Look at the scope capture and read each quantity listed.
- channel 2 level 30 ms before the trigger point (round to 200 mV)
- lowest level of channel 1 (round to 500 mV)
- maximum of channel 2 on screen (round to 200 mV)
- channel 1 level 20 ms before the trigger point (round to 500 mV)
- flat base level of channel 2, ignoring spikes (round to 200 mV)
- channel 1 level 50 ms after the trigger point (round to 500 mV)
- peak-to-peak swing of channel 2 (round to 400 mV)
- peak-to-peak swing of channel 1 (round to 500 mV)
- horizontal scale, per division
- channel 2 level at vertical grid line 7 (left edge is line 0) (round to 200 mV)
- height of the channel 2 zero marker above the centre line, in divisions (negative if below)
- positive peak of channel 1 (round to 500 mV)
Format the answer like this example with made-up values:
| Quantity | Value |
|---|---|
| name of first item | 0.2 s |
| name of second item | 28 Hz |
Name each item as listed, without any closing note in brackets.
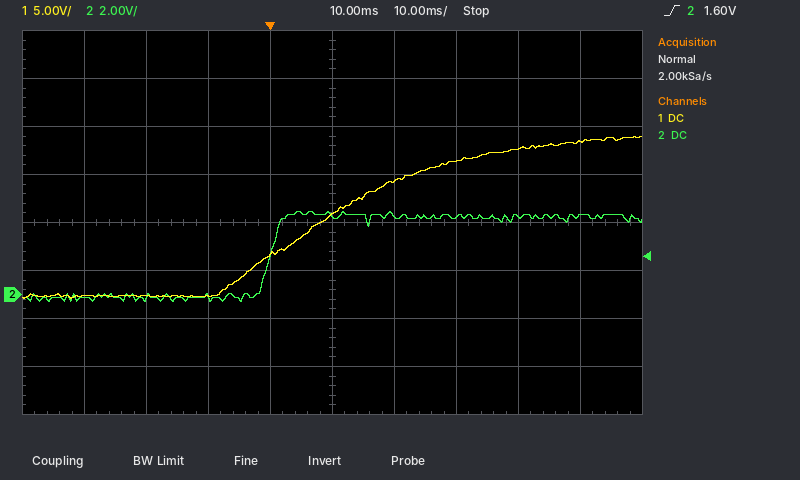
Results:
| Quantity | Value |
|---|---|
| channel 2 level 30 ms before the trigger point | -200 mV |
| lowest level of channel 1 | -500 mV |
| maximum of channel 2 on screen | 3.4 V |
| channel 1 level 20 ms before the trigger point | 0.0 V |
| flat base level of channel 2, ignoring spikes | -200 mV |
| channel 1 level 50 ms after the trigger point | 16.0 V |
| peak-to-peak swing of channel 2 | 3.6 V |
| peak-to-peak swing of channel 1 | 17.0 V |
| horizontal scale, per division | 10 ms |
| channel 2 level at vertical grid line 7 (left edge is line 0) | 3.2 V |
| height of the channel 2 zero marker above the centre line, in divisions | -1.5 div |
| positive peak of channel 1 | 16.5 V |
